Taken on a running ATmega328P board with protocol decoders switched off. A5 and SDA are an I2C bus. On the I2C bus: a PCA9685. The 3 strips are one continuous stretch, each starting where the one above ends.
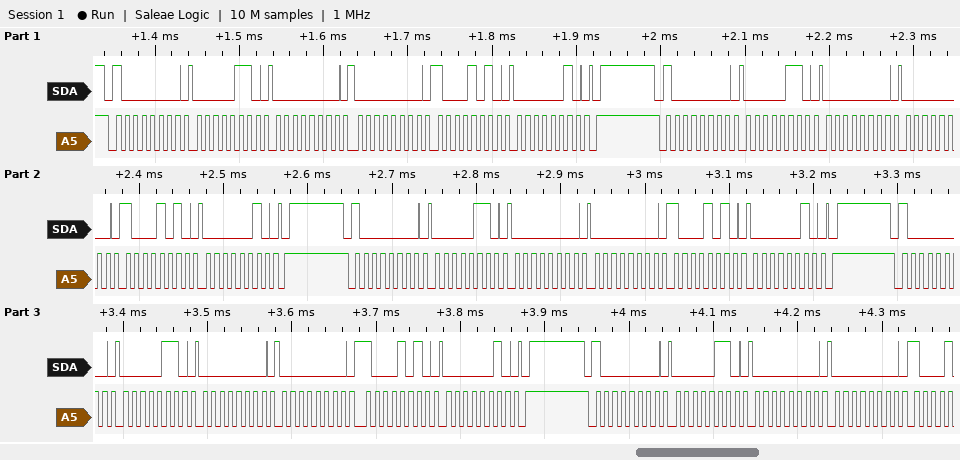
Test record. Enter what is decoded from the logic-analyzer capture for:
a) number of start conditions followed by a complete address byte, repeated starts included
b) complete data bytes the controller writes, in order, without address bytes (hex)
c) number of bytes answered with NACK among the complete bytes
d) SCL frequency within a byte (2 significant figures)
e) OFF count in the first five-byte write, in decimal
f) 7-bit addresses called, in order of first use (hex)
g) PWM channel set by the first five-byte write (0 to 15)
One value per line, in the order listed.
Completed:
5
06 00 00 8A 02 06 00 00 8A 02 06 00 00 8A 02 06 00 00 8A 02 06 00 00
0
100 kHz
650
0x40
0
